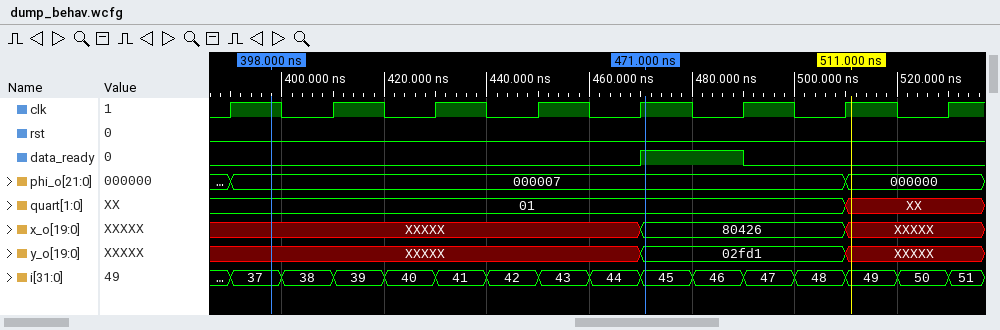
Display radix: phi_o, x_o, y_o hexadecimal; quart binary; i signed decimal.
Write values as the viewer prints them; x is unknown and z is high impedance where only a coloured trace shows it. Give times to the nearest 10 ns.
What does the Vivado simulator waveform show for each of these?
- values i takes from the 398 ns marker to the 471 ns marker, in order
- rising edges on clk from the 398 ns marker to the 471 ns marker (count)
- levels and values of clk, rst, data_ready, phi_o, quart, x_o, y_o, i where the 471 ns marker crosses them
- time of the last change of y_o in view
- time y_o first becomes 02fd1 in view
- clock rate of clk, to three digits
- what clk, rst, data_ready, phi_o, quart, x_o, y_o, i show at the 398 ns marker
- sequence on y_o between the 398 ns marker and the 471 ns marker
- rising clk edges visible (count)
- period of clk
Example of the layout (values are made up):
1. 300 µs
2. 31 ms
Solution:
1. 37, 38, 39, 40, 41, 42, 43, 44, 45
2. 4
3. clk=1, rst=0, data_ready=1, phi_o=000007, quart=01, x_o=80426, y_o=02fd1, i=45
4. 510 ns
5. 470 ns
6. 50.0 MHz
7. clk=1, rst=0, data_ready=0, phi_o=000007, quart=01, x_o=XXXXX, y_o=XXXXX, i=37
8. XXXXX, 02fd1
9. 8
10. 20 ns
